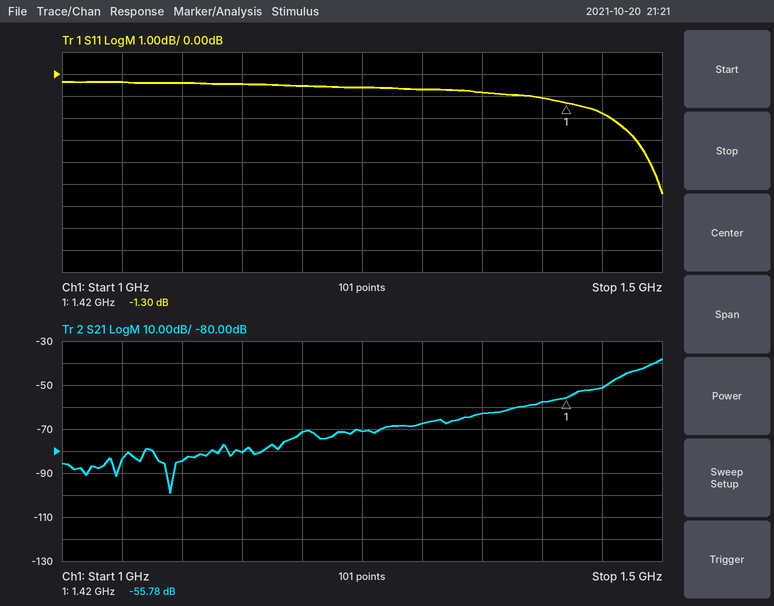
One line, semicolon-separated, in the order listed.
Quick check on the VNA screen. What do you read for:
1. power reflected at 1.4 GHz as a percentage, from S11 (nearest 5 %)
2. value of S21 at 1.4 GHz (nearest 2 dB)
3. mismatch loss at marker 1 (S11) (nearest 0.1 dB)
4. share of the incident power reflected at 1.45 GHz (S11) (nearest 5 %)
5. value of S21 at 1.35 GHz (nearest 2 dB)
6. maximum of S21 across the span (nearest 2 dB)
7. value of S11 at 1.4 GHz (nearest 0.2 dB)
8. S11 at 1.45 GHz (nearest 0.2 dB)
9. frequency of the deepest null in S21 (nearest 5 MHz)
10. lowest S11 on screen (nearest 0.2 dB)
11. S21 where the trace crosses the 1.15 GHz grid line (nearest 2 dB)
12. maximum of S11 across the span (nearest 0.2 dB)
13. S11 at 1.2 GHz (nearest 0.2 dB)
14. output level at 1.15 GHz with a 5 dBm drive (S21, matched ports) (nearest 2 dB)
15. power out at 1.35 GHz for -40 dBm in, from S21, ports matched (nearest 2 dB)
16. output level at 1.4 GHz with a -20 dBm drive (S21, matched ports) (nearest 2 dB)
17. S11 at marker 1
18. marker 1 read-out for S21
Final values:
80 %; -58 dB; 5.9 dB; 65 %; -62 dB; -38 dB; -1.0 dB; -1.8 dB; 1.090 GHz; -5.4 dB; -80 dB; -0.4 dB; -0.6 dB; -76 dBm; -102 dBm; -78 dBm; -1.30 dB; -55.78 dB
